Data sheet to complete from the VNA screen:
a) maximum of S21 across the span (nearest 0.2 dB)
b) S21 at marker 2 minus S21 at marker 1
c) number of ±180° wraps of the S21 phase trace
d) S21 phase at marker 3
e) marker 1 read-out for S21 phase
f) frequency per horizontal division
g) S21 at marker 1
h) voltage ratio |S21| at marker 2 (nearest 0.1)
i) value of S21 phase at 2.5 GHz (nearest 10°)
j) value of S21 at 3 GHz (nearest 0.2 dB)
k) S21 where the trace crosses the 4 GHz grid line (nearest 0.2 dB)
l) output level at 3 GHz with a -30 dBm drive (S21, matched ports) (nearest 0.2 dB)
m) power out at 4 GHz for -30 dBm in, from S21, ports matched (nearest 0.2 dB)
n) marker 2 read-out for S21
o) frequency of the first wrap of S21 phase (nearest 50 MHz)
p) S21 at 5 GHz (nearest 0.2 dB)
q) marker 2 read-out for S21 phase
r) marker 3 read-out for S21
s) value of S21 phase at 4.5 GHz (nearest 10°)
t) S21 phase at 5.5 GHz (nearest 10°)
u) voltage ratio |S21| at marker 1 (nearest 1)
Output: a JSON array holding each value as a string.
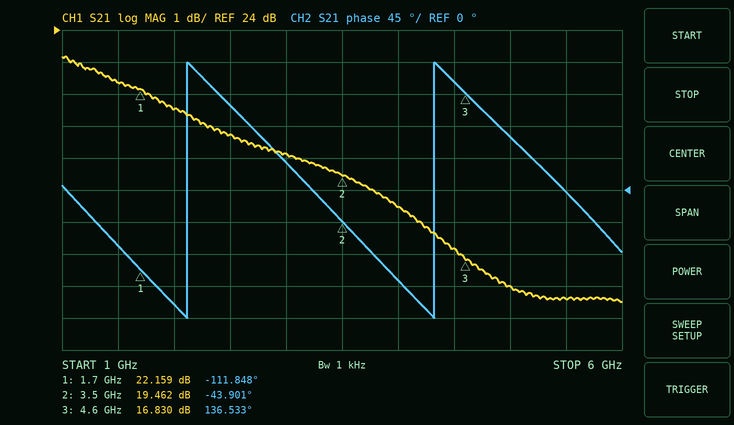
["23.2 dB", "-2.697 dB", "2", "136.533°", "-111.848°", "500 MHz", "22.159 dB", "9.4", "120°", "20.2 dB", "18.4 dB", "-9.8 dBm", "-11.6 dBm", "19.462 dB", "2.10 GHz", "16.0 dB", "-43.901°", "16.830 dB", "150°", "0°", "13"]
